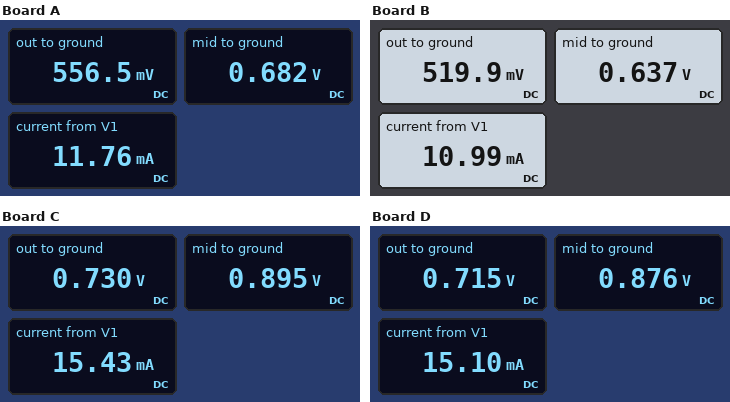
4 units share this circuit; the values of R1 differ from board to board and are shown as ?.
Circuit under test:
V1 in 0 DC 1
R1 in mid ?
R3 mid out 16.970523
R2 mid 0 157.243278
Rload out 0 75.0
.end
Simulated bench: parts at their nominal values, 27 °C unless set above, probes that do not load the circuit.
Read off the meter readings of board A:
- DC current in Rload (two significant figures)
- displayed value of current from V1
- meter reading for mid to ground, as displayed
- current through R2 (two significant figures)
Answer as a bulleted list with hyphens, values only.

- 7.4 mA
- 11.76 mA
- 0.682 V
- 4.3 mA
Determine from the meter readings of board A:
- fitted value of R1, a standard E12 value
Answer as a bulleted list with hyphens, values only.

- 27 Ω
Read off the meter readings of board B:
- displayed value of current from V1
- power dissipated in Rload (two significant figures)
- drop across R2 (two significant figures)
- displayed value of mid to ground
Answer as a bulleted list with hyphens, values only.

- 10.99 mA
- 3.6 mW
- 640 mV
- 0.637 V
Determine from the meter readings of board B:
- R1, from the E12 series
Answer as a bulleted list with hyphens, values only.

- 33 Ω
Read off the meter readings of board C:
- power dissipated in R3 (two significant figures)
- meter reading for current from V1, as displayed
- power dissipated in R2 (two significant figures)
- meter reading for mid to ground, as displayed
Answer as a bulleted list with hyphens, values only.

- 1.6 mW
- 15.43 mA
- 5.1 mW
- 0.895 V
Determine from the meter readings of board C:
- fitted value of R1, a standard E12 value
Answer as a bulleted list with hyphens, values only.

- 6.8 Ω
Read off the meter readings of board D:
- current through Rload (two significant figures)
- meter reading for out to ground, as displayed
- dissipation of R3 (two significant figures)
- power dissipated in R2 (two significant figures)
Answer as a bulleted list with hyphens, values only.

- 9.5 mA
- 0.715 V
- 1.5 mW
- 4.9 mW
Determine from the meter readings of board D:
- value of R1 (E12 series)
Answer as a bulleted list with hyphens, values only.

- 8.2 Ω
